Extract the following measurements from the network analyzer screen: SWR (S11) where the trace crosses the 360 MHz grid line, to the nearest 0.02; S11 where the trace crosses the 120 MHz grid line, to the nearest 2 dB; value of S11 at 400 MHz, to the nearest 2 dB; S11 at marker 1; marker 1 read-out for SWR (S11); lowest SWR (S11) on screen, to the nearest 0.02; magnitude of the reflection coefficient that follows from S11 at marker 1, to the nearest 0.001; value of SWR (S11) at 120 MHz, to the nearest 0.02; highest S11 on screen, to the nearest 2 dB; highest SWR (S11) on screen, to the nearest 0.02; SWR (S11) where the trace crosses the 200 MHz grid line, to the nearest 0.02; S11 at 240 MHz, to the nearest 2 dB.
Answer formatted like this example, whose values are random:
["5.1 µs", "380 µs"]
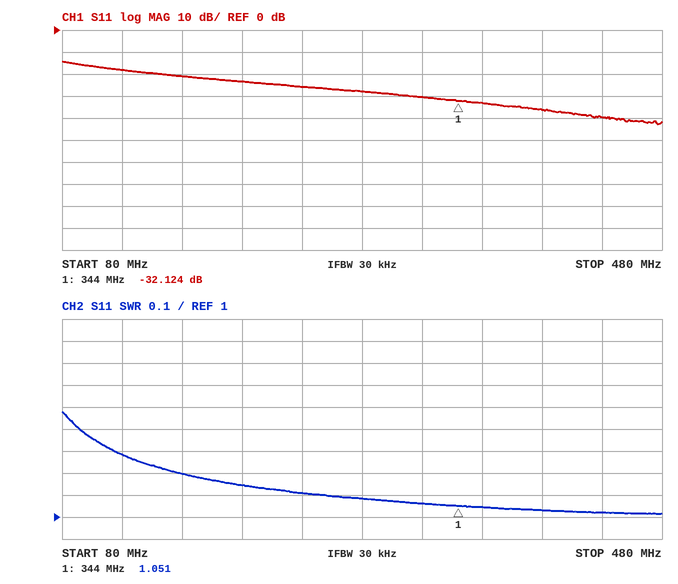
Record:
["1.04", "-18 dB", "-36 dB", "-32.124 dB", "1.051", "1.02", "0.025", "1.28", "-14 dB", "1.48", "1.14", "-26 dB"]
